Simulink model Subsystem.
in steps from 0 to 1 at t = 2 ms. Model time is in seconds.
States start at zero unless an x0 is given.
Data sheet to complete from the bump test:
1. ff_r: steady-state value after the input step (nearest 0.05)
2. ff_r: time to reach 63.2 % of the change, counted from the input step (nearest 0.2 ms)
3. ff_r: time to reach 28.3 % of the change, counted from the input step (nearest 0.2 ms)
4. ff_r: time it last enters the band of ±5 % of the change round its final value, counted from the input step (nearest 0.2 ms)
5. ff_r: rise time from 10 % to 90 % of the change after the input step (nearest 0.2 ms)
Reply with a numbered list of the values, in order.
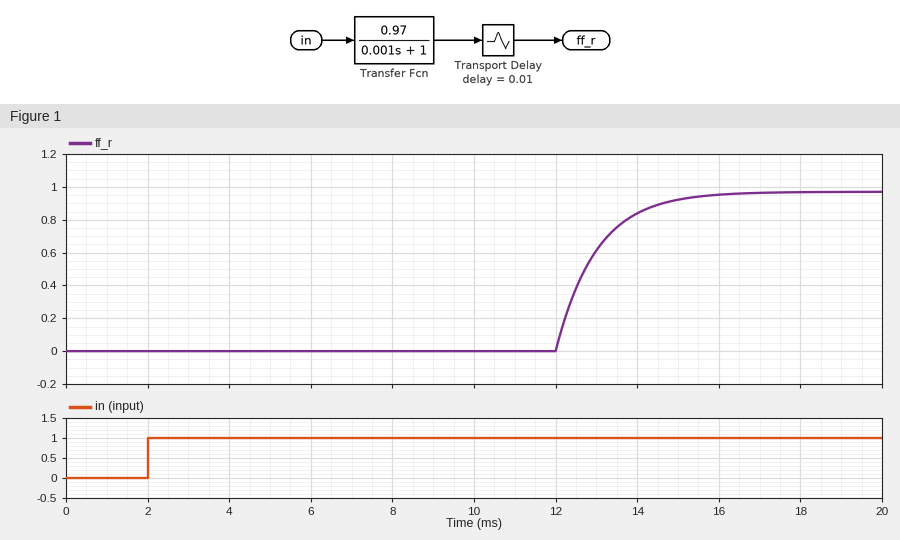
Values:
1. 0.95
2. 11.0 ms
3. 10.4 ms
4. 13.0 ms
5. 2.2 ms
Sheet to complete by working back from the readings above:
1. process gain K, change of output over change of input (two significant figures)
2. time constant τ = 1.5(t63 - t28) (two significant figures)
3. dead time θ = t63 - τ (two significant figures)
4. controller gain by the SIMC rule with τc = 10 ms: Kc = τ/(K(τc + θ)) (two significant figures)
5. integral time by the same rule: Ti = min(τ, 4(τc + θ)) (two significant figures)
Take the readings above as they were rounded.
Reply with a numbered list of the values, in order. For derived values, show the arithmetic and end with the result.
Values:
1. (0.95 - 0) / 1 = 0.95
2. 1.5 × (11 - 10.4) = 0.90 ms
3. 11 - 0.9 = 10 ms
4. 0.9 / (0.95 × (10 + 10)) = 0.047
5. min(0.9, 4 × (10 + 10)) = 0.90 ms
